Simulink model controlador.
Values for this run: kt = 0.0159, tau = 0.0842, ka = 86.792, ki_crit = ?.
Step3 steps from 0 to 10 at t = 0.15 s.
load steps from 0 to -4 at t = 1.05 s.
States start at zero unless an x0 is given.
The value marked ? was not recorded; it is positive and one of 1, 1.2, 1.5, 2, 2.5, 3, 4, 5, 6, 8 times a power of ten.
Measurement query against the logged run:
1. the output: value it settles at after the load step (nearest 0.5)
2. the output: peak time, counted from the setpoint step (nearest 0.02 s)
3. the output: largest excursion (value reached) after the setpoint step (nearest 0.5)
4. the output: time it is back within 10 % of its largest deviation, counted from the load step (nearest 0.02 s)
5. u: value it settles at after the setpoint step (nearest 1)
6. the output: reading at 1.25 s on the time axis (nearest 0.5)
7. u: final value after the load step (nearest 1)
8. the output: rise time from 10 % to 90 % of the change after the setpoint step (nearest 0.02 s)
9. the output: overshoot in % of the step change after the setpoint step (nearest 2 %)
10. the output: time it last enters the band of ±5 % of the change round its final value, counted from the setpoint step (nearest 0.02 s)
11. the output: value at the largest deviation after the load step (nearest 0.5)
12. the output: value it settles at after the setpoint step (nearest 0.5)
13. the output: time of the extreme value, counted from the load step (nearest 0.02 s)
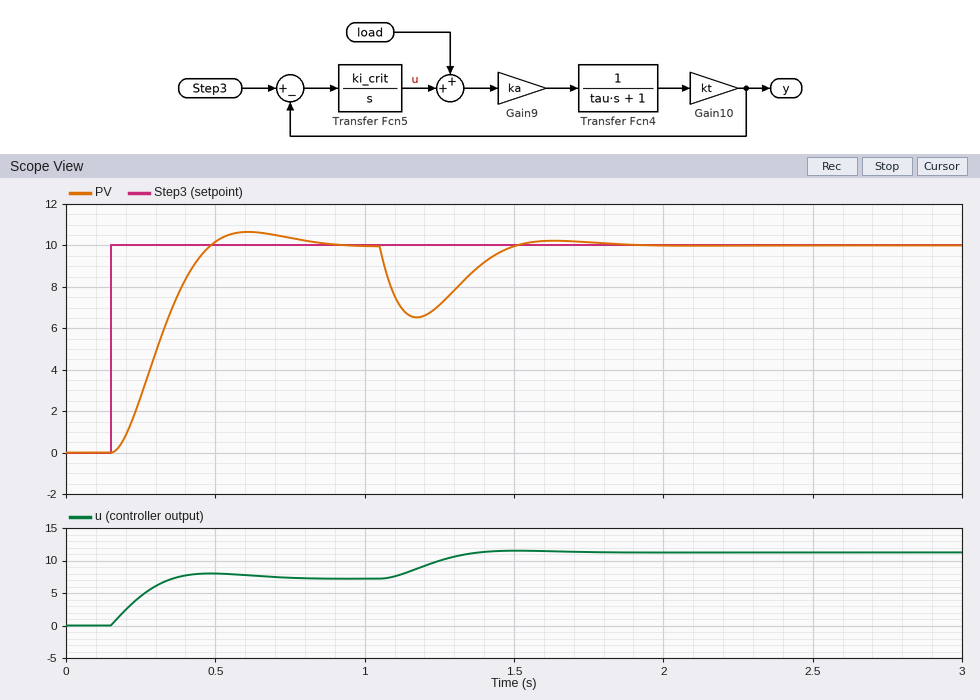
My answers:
10.0
0.46 s
10.5
0.40 s
7
7.0
11
0.22 s
6 %
0.56 s
6.5
10.0
0.12 s
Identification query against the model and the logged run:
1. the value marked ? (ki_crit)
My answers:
5
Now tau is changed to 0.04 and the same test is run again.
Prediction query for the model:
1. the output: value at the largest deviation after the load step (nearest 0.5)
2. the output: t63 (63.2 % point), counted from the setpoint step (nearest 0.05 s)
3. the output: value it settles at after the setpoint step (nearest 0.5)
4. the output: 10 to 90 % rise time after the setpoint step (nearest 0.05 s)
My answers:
6.0
0.15 s
10.0
0.25 s
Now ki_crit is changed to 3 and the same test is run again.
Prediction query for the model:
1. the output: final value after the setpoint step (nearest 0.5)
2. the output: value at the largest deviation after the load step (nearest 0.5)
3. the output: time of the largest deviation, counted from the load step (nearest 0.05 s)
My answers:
10.0
6.0
0.15 s
